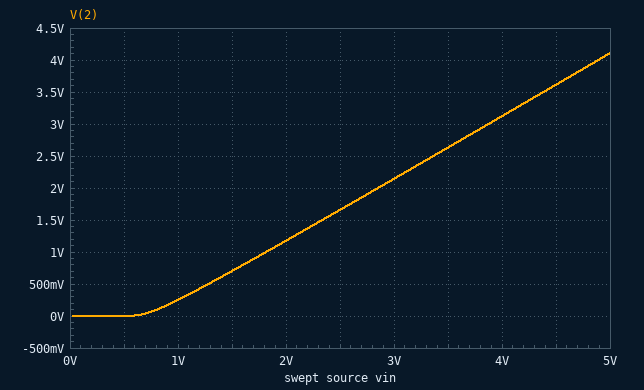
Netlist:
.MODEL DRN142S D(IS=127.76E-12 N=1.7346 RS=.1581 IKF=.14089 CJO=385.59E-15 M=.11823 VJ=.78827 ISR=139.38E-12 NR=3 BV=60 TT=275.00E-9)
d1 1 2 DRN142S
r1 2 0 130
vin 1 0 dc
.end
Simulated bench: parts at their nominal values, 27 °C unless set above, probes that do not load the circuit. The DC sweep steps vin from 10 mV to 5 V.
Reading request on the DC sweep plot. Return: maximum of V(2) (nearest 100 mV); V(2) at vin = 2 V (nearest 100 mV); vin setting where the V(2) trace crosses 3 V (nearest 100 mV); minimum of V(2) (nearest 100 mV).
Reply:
4.1 V
1.2 V
3.9 V
0 V
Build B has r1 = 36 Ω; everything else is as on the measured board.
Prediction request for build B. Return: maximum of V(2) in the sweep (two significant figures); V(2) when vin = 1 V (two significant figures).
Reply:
4.0 V
200 mV
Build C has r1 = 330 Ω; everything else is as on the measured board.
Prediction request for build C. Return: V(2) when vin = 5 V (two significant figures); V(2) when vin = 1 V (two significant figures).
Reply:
4.2 V
290 mV
